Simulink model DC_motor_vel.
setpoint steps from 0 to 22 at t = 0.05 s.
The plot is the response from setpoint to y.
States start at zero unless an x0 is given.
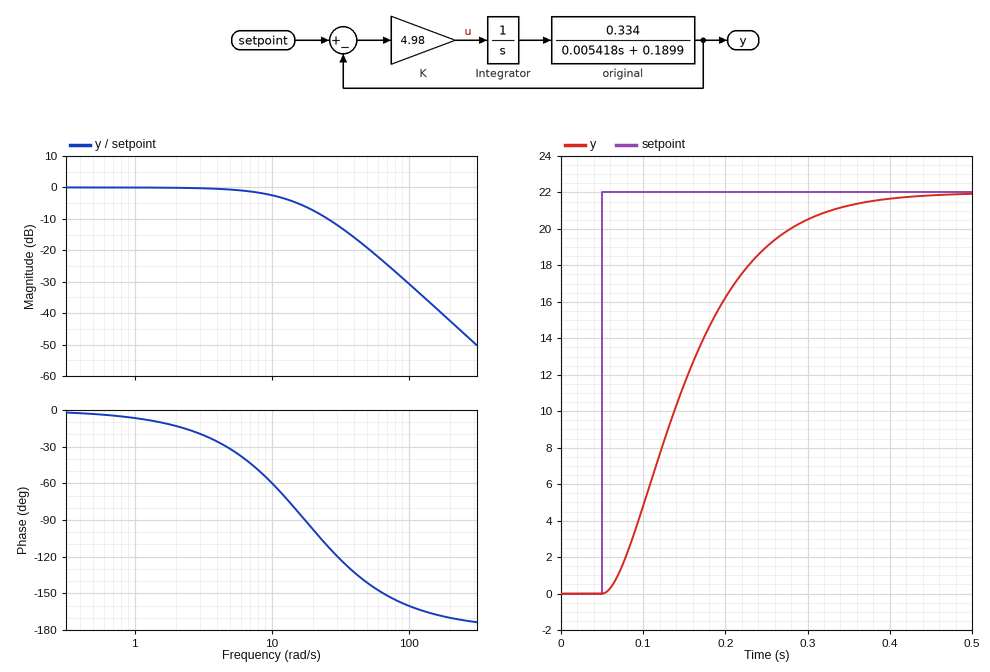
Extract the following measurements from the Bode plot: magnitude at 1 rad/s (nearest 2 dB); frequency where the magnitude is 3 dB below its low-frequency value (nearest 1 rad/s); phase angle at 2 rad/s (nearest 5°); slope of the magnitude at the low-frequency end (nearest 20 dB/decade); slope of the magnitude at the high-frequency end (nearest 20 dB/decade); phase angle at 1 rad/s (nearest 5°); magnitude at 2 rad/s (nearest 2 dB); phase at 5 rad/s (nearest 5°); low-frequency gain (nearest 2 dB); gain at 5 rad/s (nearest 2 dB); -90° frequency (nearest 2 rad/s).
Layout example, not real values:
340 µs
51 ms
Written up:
0 dB
11 rad/s
-15°
0 dB/decade
-40 dB/decade
-5°
0 dB
-30°
0 dB
0 dB
18 rad/s
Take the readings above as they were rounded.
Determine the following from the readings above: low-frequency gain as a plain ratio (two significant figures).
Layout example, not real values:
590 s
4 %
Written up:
1.0
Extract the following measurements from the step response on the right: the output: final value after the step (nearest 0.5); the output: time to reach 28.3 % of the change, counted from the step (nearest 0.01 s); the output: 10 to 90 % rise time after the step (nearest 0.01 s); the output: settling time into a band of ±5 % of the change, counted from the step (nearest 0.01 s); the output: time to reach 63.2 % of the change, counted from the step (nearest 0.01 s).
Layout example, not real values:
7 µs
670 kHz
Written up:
22.0
0.06 s
0.19 s
0.27 s
0.12 s
